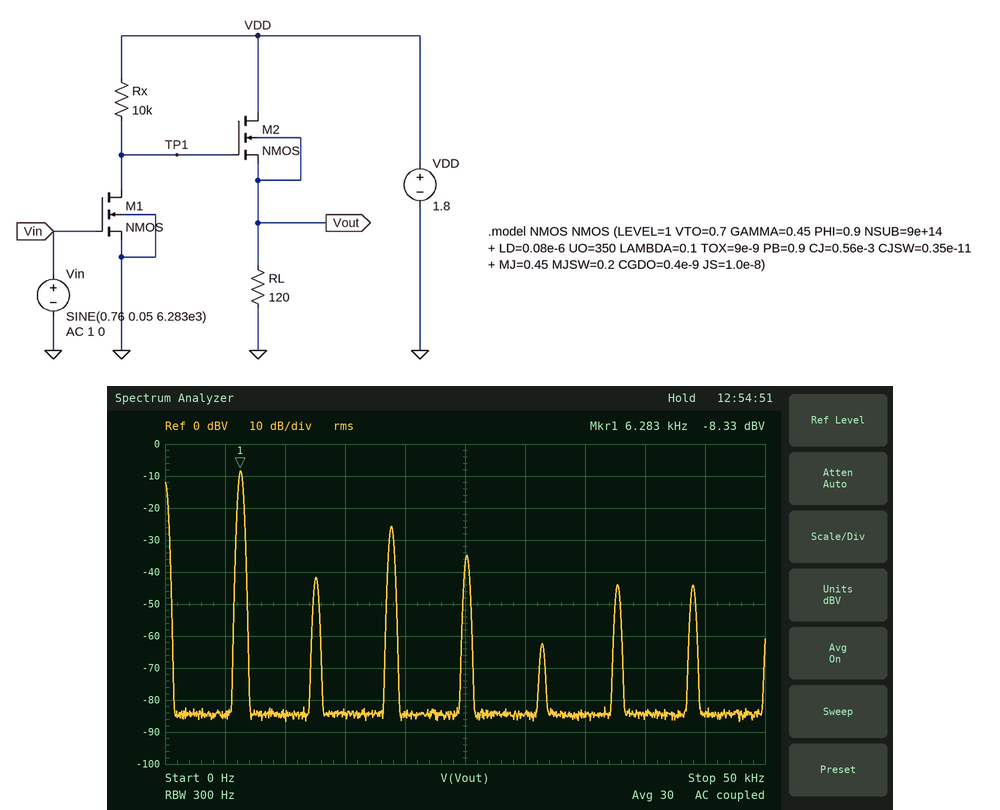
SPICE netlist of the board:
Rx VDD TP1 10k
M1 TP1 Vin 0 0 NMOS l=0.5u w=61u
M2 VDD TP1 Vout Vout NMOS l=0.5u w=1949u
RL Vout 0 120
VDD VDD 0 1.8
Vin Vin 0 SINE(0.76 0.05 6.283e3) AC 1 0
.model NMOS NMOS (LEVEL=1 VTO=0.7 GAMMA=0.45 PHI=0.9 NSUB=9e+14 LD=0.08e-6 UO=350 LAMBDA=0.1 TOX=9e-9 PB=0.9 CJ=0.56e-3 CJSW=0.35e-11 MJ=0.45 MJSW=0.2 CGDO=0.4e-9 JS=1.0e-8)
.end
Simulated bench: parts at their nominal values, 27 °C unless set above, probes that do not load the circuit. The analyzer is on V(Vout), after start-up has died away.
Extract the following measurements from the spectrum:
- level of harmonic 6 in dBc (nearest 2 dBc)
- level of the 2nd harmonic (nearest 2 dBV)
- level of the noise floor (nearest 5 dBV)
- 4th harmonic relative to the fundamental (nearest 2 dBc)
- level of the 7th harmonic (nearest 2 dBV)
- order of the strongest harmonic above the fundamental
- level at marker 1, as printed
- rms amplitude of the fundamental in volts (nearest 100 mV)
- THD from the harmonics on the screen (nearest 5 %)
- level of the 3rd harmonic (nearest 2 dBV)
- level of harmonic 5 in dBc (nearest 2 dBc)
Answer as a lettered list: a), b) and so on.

a) -36 dBc
b) -42 dBV
c) -85 dBV
d) -26 dBc
e) -44 dBV
f) 3
g) -8.33 dBV
h) 400 mV
i) 15 %
j) -26 dBV
k) -54 dBc
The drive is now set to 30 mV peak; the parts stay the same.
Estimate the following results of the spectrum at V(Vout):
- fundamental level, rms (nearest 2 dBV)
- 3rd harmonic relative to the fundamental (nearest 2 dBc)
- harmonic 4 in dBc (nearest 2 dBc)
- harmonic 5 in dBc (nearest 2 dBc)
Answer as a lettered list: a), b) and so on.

a) -10 dBV
b) -38 dBc
c) -50 dBc
d) -58 dBc
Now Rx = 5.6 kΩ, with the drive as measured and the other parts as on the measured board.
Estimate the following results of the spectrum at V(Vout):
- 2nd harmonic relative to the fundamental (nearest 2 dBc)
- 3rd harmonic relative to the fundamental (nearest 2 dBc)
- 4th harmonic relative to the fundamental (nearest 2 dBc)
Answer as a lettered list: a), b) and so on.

a) -14 dBc
b) -38 dBc
c) -54 dBc
